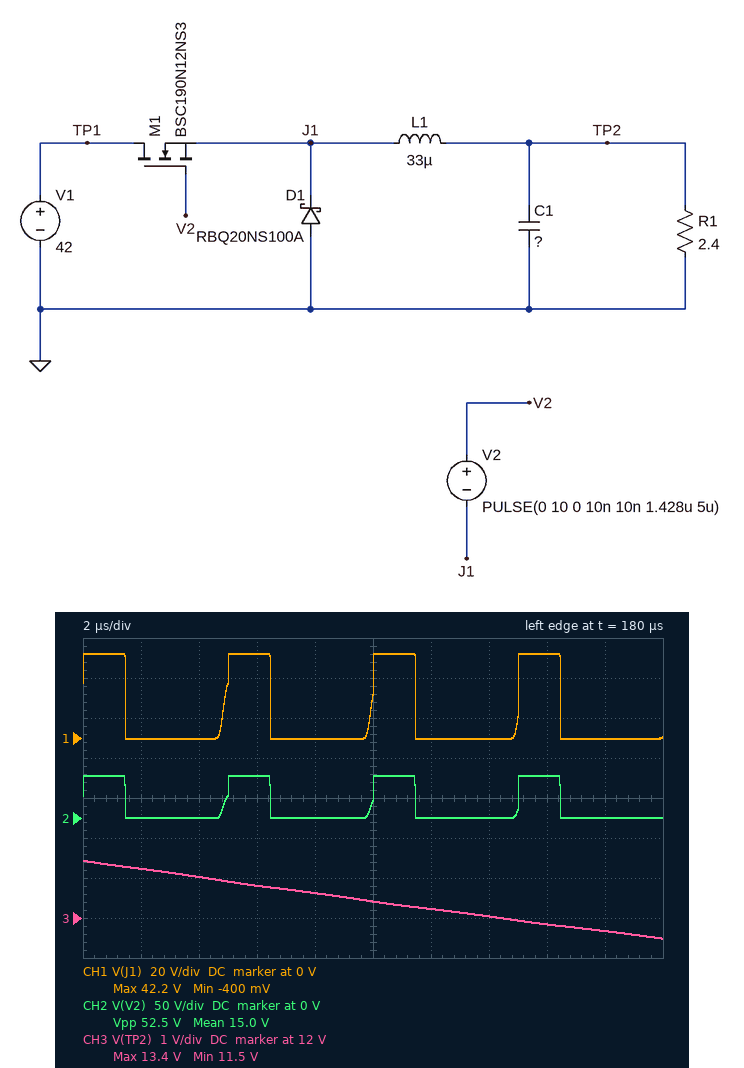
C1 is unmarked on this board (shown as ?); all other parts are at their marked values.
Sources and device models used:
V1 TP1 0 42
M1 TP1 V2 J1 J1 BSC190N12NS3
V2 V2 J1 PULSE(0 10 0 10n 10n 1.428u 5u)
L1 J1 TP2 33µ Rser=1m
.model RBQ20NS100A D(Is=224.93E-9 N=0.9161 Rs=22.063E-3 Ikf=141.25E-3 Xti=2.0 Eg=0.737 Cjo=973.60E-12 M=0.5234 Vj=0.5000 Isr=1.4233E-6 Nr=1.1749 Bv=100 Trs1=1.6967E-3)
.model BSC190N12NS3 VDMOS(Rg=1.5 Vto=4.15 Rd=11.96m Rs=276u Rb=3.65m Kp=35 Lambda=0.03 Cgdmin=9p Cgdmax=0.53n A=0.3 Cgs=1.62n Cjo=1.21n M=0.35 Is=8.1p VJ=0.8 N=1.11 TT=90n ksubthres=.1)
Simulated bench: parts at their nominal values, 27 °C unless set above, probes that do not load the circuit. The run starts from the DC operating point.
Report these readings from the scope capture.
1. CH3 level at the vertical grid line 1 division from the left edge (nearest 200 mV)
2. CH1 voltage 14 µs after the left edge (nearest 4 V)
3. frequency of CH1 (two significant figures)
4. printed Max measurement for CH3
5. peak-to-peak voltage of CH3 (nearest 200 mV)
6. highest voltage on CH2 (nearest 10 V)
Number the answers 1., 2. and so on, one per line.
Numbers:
1. 13.2 V
2. 0 V
3. 200 kHz
4. 13.4 V
5. 2.0 V
6. 50 V
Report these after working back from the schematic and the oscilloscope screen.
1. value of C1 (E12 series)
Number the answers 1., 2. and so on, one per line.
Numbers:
1. 47 µF
